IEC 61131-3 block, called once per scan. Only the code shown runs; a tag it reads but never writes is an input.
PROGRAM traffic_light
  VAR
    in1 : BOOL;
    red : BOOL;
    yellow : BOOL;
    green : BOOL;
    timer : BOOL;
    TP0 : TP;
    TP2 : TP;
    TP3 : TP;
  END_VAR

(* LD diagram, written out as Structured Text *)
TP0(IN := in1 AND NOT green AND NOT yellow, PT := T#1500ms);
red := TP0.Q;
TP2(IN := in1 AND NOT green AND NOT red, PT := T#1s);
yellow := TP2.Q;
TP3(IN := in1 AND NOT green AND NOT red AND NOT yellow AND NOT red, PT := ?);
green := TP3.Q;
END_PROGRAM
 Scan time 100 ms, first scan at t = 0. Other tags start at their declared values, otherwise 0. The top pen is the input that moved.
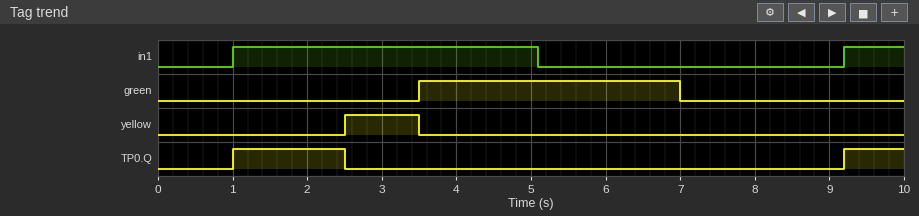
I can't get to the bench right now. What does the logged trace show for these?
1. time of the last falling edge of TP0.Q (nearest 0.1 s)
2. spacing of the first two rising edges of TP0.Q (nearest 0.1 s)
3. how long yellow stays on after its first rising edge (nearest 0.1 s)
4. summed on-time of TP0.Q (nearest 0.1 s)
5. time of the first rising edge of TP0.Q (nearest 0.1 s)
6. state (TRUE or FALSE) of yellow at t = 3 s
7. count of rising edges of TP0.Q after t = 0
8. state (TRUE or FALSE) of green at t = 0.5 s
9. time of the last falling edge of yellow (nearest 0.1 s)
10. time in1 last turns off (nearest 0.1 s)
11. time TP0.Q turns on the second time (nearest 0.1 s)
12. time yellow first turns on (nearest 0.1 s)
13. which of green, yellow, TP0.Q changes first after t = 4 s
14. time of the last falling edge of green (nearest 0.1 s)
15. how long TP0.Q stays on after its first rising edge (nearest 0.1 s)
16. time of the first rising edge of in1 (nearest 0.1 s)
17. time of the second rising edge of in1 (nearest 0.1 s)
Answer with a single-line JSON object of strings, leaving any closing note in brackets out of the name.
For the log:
{"time of the last falling edge of TP0.Q": "2.5 s", "spacing of the first two rising edges of TP0.Q": "8.2 s", "how long yellow stays on after its first rising edge": "1.0 s", "summed on-time of TP0.Q": "2.3 s", "time of the first rising edge of TP0.Q": "1.0 s", "state (TRUE or FALSE) of yellow at t = 3 s": "TRUE", "count of rising edges of TP0.Q after t = 0": "2", "state (TRUE or FALSE) of green at t = 0.5 s": "FALSE", "time of the last falling edge of yellow": "3.5 s", "time in1 last turns off": "5.1 s", "time TP0.Q turns on the second time": "9.2 s", "time yellow first turns on": "2.5 s", "which of green, yellow, TP0.Q changes first after t = 4 s": "green", "time of the last falling edge of green": "7.0 s", "how long TP0.Q stays on after its first rising edge": "1.5 s", "time of the first rising edge of in1": "1.0 s", "time of the second rising edge of in1": "9.2 s"}
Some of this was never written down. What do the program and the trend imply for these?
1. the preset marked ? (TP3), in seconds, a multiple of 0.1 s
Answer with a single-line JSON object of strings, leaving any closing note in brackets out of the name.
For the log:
{"the preset marked ? (TP3), in seconds, a multiple of 0.1 s": "3.5 s"}
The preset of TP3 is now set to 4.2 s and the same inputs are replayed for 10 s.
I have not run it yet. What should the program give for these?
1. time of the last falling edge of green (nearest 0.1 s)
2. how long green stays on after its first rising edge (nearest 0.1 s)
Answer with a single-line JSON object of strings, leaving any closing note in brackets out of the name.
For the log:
{"time of the last falling edge of green": "7.7 s", "how long green stays on after its first rising edge": "4.2 s"}
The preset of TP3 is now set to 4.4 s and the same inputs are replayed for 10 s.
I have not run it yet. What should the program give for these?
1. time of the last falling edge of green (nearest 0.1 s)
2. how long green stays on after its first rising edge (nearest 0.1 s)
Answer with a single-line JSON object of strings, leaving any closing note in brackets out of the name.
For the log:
{"time of the last falling edge of green": "7.9 s", "how long green stays on after its first rising edge": "4.4 s"}
